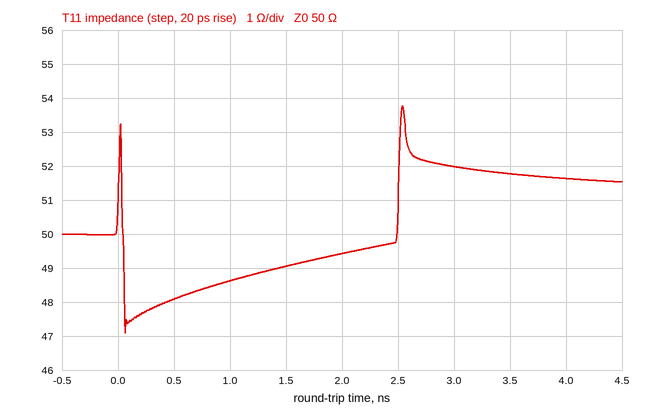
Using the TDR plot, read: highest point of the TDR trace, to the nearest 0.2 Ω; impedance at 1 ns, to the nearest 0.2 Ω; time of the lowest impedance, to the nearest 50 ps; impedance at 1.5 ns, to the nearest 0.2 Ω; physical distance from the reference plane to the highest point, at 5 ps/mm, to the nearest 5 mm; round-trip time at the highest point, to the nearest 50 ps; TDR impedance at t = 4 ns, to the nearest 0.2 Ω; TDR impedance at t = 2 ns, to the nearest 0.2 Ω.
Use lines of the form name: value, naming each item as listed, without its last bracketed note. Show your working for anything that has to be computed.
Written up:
highest point of the TDR trace, to the nearest 0.2 Ω: 53.8 Ω
impedance at 1 ns, to the nearest 0.2 Ω: 48.6 Ω
time of the lowest impedance, to the nearest 50 ps: 50 ps
impedance at 1.5 ns, to the nearest 0.2 Ω: 49.0 Ω
physical distance from the reference plane to the highest point, at 5 ps/mm, to the nearest 5 mm: 2.55 ns / 2 / 5 ps/mm ≈ 255 mm
round-trip time at the highest point, to the nearest 50 ps: 2.55 ns
TDR impedance at t = 4 ns, to the nearest 0.2 Ω: 51.6 Ω
TDR impedance at t = 2 ns, to the nearest 0.2 Ω: 49.4 Ω
